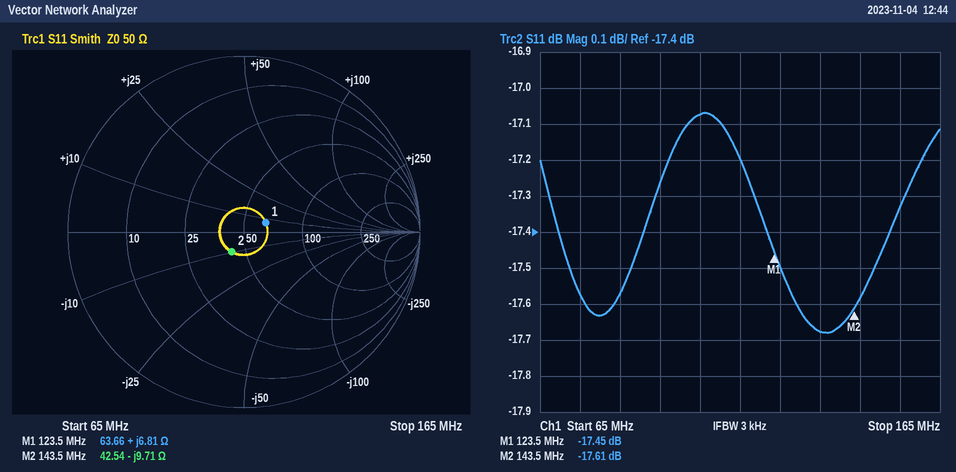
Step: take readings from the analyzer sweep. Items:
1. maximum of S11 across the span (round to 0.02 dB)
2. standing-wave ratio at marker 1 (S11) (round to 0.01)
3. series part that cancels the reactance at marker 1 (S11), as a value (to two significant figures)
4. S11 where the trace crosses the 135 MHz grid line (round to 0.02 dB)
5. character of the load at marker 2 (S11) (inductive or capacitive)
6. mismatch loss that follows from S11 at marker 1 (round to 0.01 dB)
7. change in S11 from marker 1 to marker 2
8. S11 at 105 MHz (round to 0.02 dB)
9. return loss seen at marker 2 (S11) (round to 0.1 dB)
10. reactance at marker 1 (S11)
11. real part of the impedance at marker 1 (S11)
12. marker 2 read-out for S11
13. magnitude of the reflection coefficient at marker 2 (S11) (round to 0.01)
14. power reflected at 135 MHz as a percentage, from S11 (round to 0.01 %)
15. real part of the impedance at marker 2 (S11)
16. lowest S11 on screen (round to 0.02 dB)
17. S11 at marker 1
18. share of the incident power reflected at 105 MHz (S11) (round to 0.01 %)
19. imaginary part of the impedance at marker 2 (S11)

-17.06 dB
1.31
190 pF
-17.68 dB
capacitive
0.08 dB
-0.16 dB
-17.08 dB
17.6 dB
+6.81 Ω
63.66 Ω
-17.61 dB
0.13
1.71 %
42.54 Ω
-17.68 dB
-17.45 dB
1.96 %
-9.71 Ω
